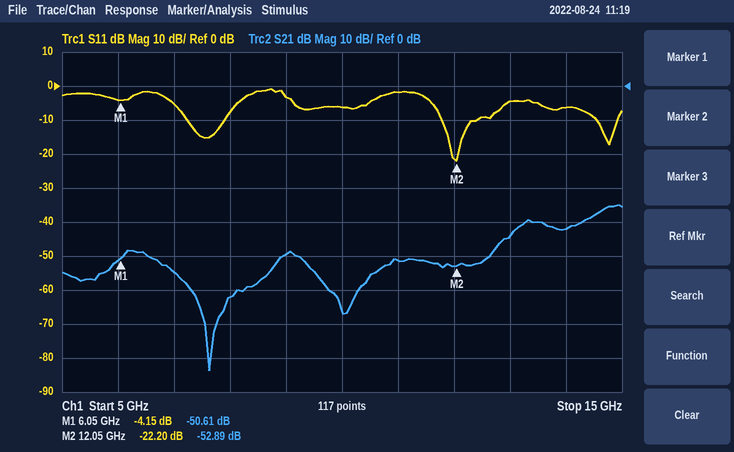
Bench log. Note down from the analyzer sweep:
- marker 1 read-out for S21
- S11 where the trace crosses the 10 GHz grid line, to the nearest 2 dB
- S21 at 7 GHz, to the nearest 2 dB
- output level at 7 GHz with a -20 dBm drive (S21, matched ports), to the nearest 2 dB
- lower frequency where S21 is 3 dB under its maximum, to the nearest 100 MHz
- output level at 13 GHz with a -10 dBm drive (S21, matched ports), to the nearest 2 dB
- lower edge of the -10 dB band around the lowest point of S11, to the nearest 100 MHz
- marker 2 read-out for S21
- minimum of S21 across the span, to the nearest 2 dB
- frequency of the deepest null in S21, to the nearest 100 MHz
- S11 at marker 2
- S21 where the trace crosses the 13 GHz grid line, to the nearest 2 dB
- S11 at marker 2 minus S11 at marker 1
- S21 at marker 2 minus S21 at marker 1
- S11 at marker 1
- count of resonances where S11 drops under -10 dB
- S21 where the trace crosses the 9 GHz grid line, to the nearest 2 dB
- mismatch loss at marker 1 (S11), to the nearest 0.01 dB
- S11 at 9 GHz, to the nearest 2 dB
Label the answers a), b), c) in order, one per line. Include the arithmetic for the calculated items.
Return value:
a) -50.61 dB
b) -6 dB
c) -54 dB
d) -20 dBm + (-54 dB) = -74 dBm
e) 14.5 GHz
f) -10 dBm + (-44 dB) = -54 dBm
g) 11.8 GHz
h) -52.89 dB
i) -84 dB
j) 7.6 GHz
k) -22.20 dB
l) -44 dB
m) -22.2 − (-4.15) = -18.05 dB
n) -52.89 − (-50.61) = -2.28 dB
o) -4.15 dB
p) 3
q) -50 dB
r) −10 log10(1 − 10^(-4.15/10)) ≈ 2.11 dB
s) -4 dB
